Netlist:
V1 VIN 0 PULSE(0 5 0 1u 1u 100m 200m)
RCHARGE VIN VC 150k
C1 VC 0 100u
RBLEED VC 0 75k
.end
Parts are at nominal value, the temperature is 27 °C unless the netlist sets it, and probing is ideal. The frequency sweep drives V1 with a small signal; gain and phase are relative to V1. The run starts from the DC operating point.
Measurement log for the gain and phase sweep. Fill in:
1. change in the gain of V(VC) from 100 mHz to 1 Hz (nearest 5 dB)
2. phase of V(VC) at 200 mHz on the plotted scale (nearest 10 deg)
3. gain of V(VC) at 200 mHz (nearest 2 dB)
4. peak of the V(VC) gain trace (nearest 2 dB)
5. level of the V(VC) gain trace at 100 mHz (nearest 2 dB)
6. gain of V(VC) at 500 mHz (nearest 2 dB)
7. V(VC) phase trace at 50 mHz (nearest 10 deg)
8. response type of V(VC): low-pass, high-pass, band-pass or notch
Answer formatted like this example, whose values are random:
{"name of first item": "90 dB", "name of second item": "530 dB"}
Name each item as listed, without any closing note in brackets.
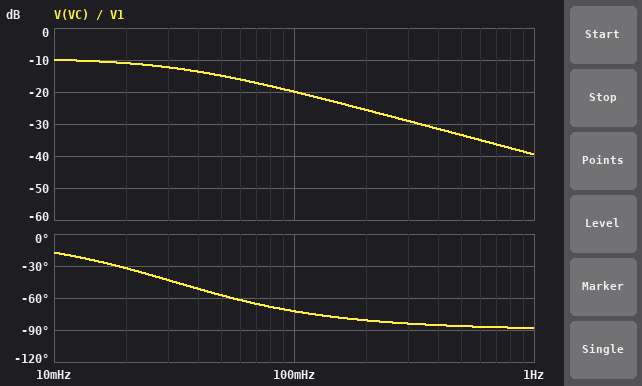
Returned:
{"change in the gain of V(VC) from 100 mHz to 1 Hz": "-20 dB", "phase of V(VC) at 200 mHz on the plotted scale": "-80 deg", "gain of V(VC) at 200 mHz": "-26 dB", "peak of the V(VC) gain trace": "-10 dB", "level of the V(VC) gain trace at 100 mHz": "-20 dB", "gain of V(VC) at 500 mHz": "-34 dB", "V(VC) phase trace at 50 mHz": "-60 deg", "response type of V(VC): low-pass, high-pass, band-pass or notch": "low-pass"}
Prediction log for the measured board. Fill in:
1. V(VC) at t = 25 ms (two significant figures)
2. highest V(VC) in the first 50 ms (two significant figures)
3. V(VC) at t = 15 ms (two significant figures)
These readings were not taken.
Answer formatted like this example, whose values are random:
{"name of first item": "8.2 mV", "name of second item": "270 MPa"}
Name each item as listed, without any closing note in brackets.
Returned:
{"V(VC) at t = 25 ms": "8.3 mV", "highest V(VC) in the first 50 ms": "17 mV", "V(VC) at t = 15 ms": "5.0 mV"}
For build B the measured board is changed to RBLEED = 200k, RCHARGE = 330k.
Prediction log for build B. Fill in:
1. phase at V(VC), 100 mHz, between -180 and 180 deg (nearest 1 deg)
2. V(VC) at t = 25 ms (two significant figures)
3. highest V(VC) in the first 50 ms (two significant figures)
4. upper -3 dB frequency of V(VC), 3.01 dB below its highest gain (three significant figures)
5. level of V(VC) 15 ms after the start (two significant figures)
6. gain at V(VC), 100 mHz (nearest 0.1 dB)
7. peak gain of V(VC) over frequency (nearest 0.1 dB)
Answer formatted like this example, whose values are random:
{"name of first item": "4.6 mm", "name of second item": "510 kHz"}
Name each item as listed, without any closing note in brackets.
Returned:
{"phase at V(VC), 100 mHz, between -180 and 180 deg": "-83 deg", "V(VC) at t = 25 ms": "3.8 mV", "highest V(VC) in the first 50 ms": "7.6 mV", "upper -3 dB frequency of V(VC), 3.01 dB below its highest gain": "12.8 mHz", "level of V(VC) 15 ms after the start": "2.3 mV", "gain at V(VC), 100 mHz": "-26.4 dB", "peak gain of V(VC) over frequency": "-8.5 dB"}
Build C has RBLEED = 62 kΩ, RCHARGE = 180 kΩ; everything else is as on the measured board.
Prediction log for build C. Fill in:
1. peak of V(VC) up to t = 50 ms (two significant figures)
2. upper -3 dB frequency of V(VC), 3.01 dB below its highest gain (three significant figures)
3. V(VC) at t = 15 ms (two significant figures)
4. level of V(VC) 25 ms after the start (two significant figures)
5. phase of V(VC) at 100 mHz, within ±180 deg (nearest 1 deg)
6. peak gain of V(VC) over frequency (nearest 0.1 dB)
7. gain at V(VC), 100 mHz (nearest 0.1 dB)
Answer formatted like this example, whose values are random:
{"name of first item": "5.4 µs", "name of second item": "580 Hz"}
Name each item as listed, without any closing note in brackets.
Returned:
{"peak of V(VC) up to t = 50 ms": "14 mV", "upper -3 dB frequency of V(VC), 3.01 dB below its highest gain": "34.5 mHz", "V(VC) at t = 15 ms": "4.2 mV", "level of V(VC) 25 ms after the start": "6.9 mV", "phase of V(VC) at 100 mHz, within ±180 deg": "-71 deg", "peak gain of V(VC) over frequency": "-11.8 dB", "gain at V(VC), 100 mHz": "-21.6 dB"}
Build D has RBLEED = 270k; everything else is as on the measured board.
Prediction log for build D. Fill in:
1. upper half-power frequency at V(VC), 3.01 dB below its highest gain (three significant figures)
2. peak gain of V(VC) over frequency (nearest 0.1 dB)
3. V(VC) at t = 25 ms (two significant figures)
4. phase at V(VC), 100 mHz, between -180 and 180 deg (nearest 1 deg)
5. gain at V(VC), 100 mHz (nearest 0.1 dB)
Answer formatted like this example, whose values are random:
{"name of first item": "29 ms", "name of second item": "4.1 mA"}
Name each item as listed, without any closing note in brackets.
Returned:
{"upper half-power frequency at V(VC), 3.01 dB below its highest gain": "16.5 mHz", "peak gain of V(VC) over frequency": "-3.8 dB", "V(VC) at t = 25 ms": "8.3 mV", "phase at V(VC), 100 mHz, between -180 and 180 deg": "-81 deg", "gain at V(VC), 100 mHz": "-19.6 dB"}
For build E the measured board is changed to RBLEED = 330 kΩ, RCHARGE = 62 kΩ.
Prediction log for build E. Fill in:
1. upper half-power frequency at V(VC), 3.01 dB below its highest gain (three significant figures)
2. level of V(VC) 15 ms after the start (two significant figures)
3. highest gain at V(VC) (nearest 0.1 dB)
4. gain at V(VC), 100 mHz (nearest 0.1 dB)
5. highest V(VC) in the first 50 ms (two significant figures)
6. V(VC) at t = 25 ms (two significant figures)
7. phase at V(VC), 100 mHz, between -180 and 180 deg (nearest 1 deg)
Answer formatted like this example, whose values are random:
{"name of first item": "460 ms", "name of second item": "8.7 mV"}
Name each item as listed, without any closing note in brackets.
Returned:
{"upper half-power frequency at V(VC), 3.01 dB below its highest gain": "30.5 mHz", "level of V(VC) 15 ms after the start": "12 mV", "highest gain at V(VC)": "-1.5 dB", "gain at V(VC), 100 mHz": "-12.2 dB", "highest V(VC) in the first 50 ms": "40 mV", "V(VC) at t = 25 ms": "20 mV", "phase at V(VC), 100 mHz, between -180 and 180 deg": "-73 deg"}
